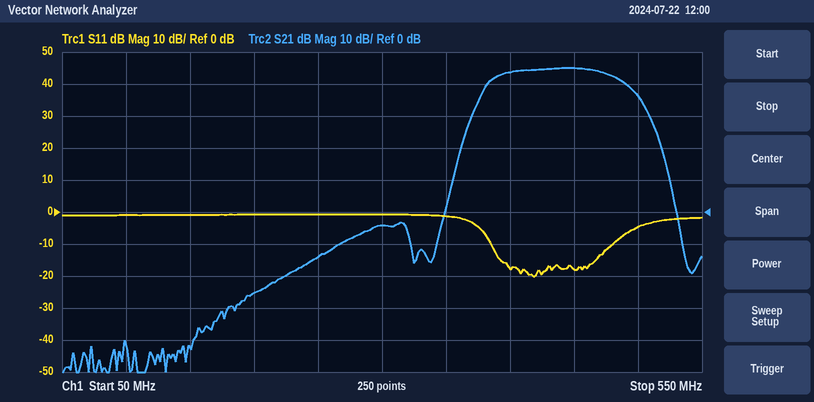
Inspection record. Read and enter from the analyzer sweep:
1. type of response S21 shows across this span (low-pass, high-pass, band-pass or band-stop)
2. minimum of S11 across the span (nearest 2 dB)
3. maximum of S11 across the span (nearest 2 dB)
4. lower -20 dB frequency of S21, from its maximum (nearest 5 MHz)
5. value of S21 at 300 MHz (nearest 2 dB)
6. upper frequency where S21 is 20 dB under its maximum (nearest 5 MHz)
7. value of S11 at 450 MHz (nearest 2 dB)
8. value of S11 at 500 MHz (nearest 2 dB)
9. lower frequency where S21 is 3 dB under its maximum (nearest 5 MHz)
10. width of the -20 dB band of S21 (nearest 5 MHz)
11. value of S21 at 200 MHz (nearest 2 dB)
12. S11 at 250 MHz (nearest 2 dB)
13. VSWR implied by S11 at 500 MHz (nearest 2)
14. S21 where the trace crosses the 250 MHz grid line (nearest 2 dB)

band-pass
-20 dB
0 dB
365 MHz
-4 dB
515 MHz
-18 dB
-4 dB
390 MHz
150 MHz
-26 dB
0 dB
4
-14 dB
